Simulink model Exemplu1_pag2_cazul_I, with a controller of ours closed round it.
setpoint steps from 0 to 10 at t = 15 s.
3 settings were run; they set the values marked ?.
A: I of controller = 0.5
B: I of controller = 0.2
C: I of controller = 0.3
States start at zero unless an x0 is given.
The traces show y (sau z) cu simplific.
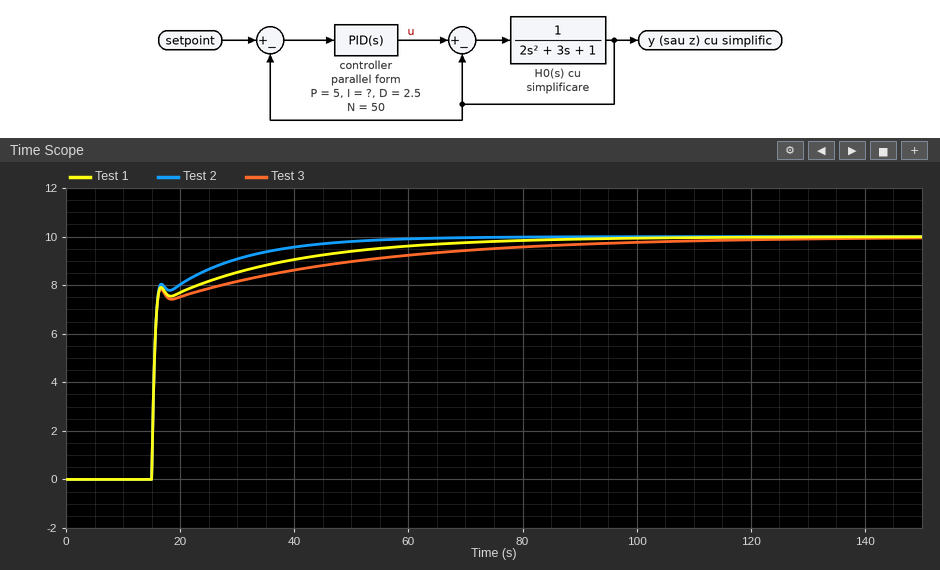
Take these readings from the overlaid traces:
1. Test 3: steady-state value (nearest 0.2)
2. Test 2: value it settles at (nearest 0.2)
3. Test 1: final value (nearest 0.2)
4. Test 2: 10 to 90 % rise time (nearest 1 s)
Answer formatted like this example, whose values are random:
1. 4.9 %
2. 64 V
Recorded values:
1. 10.0
2. 10.0
3. 10.0
4. 14 s
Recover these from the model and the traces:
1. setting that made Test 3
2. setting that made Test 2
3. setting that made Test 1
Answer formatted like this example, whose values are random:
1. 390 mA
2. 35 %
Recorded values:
1. B
2. A
3. C
